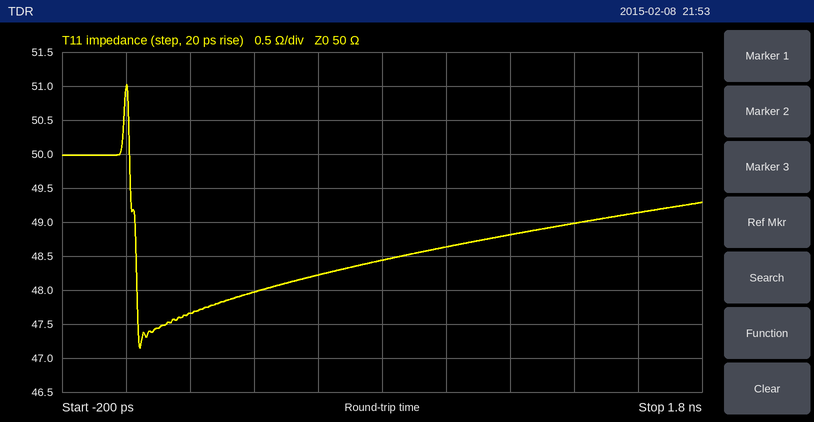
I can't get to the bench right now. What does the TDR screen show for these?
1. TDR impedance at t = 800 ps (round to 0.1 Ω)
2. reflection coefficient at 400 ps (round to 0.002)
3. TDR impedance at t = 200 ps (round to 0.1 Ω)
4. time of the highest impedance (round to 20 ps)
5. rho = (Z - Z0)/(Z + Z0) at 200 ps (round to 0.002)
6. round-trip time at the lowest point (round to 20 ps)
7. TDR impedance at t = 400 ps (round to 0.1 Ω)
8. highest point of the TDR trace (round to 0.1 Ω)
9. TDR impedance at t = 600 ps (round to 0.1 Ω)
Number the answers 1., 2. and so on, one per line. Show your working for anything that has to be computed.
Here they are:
1. 48.4 Ω
2. (48 − 50)/(48 + 50) ≈ -0.020
3. 47.7 Ω
4. 0 ps
5. (47.7 − 50)/(47.7 + 50) ≈ -0.024
6. 40 ps
7. 48.0 Ω
8. 51.0 Ω
9. 48.2 Ω
